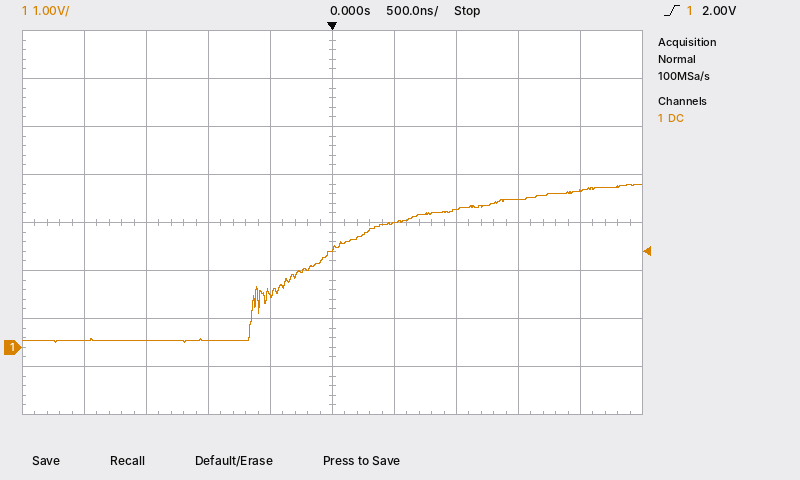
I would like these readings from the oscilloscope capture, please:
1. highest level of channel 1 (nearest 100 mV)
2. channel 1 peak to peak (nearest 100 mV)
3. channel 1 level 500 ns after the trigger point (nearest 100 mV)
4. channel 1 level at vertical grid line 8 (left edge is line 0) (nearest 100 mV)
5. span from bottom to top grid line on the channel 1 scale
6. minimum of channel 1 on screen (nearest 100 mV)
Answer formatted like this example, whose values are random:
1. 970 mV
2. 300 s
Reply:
1. 3.4 V
2. 3.3 V
3. 2.6 V
4. 3.1 V
5. 8 V
6. 100 mV
